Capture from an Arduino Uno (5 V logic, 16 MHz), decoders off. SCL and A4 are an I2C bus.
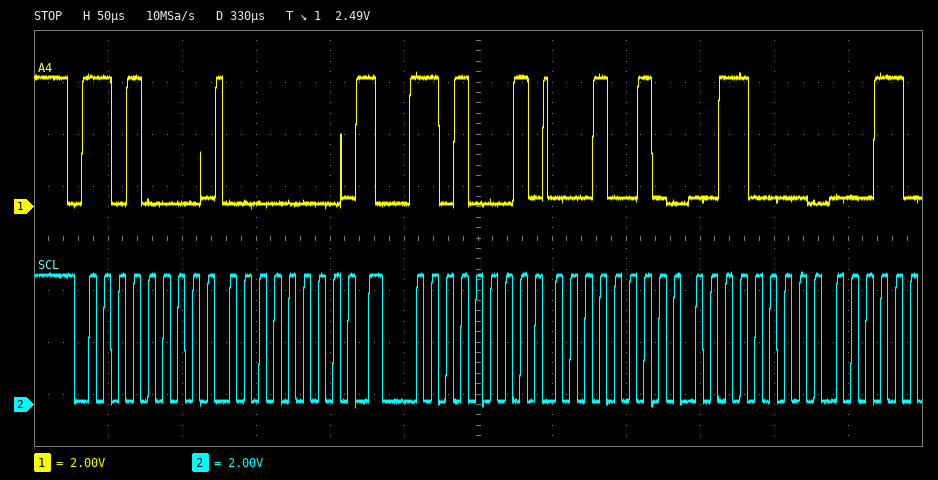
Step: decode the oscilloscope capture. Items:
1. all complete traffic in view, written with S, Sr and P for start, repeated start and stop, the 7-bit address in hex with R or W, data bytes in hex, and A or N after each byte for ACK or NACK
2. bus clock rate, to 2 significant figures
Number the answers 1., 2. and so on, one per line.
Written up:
1. S 68W A 00 A Sr 68R A 12 A 30 A
2. 100 kHz
